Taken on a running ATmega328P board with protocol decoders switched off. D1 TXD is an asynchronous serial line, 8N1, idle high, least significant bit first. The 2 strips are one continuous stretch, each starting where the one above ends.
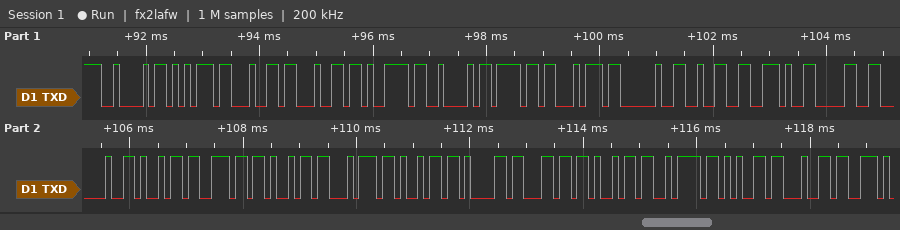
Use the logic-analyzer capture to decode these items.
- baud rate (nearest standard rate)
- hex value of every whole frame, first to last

9600 baud
0x42 0x75 0x64 0x64 0x79 0x42 0x6F 0x74 0x20 0x32 0x2E 0x30 0x20 0x69 0x6E 0x69 0x74 0x69 0x61 0x6C 0x69 0x7A 0x65 0x64
